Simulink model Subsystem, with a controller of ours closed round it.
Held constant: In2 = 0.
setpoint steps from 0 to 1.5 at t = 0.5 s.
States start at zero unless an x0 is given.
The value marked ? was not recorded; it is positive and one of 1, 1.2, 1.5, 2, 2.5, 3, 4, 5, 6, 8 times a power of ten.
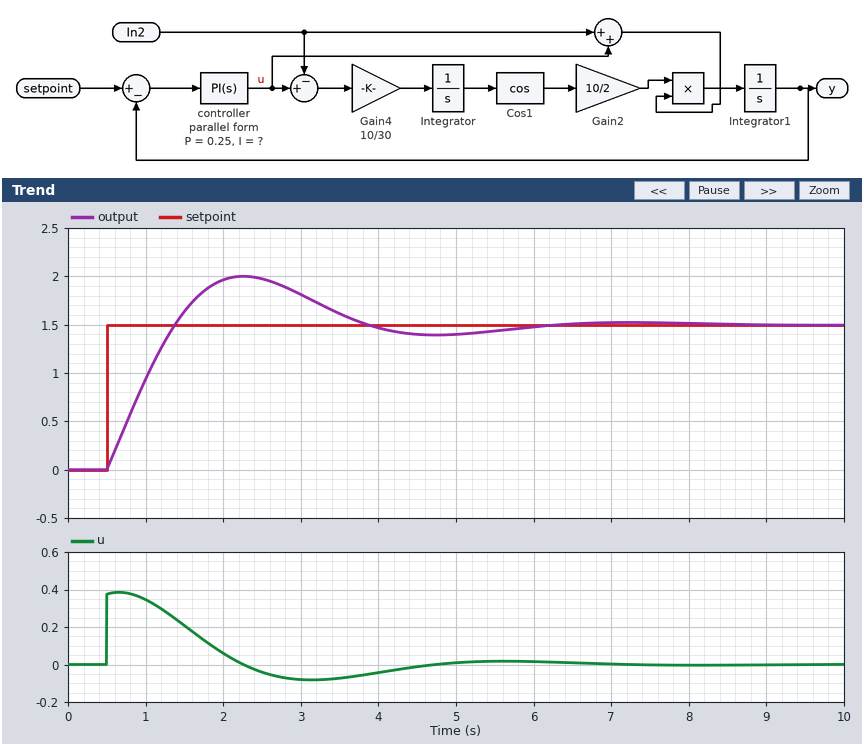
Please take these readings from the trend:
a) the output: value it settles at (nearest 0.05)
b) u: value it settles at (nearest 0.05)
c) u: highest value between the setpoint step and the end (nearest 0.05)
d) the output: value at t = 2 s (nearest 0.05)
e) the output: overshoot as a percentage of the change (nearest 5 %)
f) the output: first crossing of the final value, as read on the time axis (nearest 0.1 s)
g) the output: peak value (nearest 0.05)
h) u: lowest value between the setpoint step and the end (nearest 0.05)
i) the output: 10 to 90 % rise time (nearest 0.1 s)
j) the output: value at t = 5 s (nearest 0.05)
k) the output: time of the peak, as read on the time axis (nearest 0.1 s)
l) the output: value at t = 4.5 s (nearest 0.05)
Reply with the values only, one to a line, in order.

1.50
0.00
0.40
1.95
35 %
1.4 s
2.00
-0.10
0.7 s
1.40
2.3 s
1.40
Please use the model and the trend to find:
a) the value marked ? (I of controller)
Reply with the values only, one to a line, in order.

0.4
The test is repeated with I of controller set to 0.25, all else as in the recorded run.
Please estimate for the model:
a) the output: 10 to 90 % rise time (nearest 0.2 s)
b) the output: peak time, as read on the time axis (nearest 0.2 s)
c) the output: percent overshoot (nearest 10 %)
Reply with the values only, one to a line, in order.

0.8 s
2.6 s
30 %
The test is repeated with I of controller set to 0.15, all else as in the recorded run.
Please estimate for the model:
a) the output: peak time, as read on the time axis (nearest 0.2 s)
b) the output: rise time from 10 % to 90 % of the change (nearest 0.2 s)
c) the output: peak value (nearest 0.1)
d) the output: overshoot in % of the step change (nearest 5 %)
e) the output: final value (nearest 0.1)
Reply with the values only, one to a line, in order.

3.0 s
1.0 s
1.8
20 %
1.5
